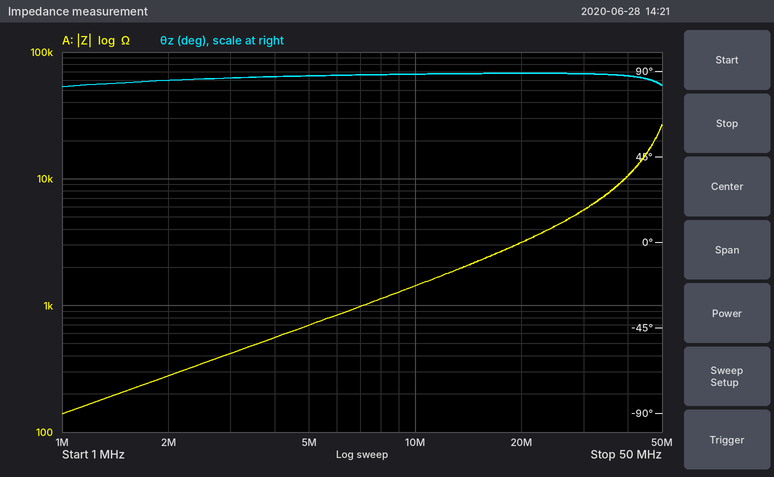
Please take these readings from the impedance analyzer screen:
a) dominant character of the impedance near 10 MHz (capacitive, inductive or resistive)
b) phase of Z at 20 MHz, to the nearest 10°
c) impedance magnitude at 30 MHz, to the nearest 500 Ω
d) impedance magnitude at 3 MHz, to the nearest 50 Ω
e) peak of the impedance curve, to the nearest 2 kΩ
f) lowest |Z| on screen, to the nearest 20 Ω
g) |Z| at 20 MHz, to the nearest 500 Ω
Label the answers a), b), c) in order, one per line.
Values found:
a) inductive
b) 90°
c) 5.5 kΩ
d) 400 Ω
e) 26 kΩ
f) 140 Ω
g) 3.0 kΩ
